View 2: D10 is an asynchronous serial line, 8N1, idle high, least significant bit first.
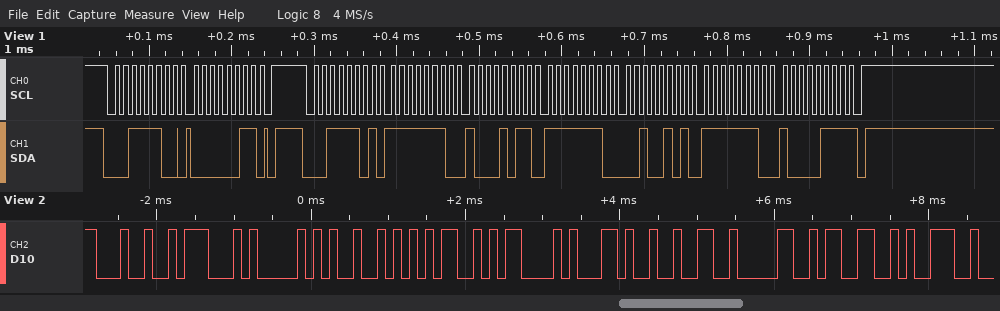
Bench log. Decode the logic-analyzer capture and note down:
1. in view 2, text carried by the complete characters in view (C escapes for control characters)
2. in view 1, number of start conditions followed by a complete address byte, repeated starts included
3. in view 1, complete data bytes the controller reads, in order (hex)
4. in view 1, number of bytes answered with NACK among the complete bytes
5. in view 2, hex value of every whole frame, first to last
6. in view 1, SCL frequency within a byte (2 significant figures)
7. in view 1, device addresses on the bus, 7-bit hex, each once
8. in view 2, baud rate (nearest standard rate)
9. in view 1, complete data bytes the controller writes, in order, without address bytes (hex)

"$GPRMC,2039"
2
FE 8B FE 25 FE 87
1
24 47 50 52 4D 43 2C 32 30 33 39
100 kHz
0x1E
9600 baud
03
